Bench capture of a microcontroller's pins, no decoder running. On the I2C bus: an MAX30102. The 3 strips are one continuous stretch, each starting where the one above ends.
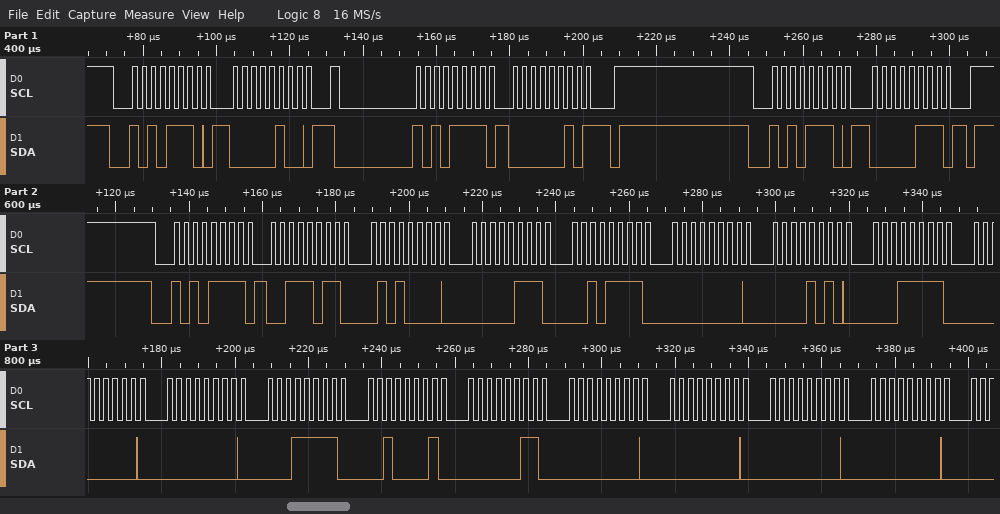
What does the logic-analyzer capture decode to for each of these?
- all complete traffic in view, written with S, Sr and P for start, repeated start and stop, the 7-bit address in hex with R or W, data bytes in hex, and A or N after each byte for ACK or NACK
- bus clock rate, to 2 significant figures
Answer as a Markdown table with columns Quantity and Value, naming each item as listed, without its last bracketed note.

| Quantity | Value |
|---|---|
| all complete traffic in view, written with S, Sr and P for start, repeated start and stop, the 7-bit address in hex with R or W, data bytes in hex, and A or N after each byte for ACK or NACK | S 57W A 04 A Sr 57R A 02 N P S 57W A 07 A P S 57R A 3B A 50 A 07 A 2F A 00 A 0A A 1F A 00 A 00 A 1F A 21 A 03 A 00 A 00 A 00 A 00 A |
| bus clock rate, to 2 significant figures | 400 kHz |
